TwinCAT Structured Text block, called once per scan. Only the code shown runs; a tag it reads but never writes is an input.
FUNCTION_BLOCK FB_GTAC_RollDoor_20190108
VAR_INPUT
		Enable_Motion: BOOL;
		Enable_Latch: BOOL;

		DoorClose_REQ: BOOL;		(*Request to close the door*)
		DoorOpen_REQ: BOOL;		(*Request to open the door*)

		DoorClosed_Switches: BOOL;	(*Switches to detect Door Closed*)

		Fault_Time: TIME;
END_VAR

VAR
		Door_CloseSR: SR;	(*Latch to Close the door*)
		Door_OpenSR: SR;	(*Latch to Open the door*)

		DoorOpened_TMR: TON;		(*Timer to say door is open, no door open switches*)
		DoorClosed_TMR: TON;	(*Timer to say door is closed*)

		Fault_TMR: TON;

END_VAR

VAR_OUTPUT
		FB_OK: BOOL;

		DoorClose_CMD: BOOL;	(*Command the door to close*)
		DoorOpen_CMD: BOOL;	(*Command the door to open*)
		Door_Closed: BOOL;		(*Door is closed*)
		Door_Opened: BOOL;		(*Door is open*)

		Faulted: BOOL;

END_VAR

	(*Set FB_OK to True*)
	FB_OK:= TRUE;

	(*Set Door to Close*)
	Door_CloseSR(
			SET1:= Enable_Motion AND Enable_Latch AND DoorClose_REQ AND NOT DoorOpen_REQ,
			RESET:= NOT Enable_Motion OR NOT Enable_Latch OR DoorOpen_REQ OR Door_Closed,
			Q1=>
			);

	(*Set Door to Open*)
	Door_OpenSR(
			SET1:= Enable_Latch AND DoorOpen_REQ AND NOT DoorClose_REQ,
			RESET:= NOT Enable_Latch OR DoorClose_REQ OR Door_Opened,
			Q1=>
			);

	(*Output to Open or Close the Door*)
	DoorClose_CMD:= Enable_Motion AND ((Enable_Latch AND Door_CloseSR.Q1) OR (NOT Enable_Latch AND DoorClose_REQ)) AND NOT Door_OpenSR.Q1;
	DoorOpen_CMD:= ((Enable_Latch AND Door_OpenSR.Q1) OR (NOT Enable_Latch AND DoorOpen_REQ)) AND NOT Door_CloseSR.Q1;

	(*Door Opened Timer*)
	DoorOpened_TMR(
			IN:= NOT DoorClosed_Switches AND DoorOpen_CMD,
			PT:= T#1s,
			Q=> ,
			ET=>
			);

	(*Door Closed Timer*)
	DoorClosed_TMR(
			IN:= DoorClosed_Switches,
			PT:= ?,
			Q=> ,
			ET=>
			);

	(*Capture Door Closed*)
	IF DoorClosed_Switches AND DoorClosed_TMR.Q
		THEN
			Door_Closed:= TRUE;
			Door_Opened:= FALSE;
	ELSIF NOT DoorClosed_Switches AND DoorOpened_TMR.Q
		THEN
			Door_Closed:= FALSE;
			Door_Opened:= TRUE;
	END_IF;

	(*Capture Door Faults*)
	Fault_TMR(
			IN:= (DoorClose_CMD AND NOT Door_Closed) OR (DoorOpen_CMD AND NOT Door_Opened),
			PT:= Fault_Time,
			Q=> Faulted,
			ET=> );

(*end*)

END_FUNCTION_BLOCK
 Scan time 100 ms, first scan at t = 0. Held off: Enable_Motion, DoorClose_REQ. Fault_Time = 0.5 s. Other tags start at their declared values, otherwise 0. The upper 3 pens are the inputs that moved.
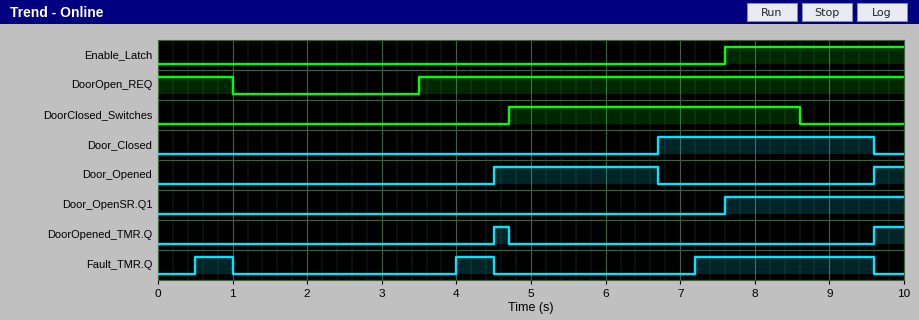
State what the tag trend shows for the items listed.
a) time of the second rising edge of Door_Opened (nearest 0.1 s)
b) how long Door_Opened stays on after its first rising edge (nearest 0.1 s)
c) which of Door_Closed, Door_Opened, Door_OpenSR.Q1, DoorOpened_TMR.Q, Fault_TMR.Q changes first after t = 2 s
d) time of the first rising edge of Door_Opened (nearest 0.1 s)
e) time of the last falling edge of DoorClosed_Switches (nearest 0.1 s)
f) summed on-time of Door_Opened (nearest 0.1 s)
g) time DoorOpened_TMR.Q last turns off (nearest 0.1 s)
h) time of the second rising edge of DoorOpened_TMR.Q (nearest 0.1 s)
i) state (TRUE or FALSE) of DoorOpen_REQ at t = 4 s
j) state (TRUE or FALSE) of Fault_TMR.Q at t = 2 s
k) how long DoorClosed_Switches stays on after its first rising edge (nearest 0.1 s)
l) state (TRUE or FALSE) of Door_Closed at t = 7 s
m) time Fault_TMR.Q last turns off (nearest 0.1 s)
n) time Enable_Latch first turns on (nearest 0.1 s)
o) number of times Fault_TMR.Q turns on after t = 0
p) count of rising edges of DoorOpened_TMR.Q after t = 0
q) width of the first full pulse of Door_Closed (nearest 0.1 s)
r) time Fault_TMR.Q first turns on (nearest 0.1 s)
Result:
9.6 s
2.2 s
Fault_TMR.Q
4.5 s
8.6 s
2.6 s
4.7 s
9.6 s
TRUE
FALSE
3.9 s
TRUE
9.6 s
7.6 s
3
2
2.9 s
0.5 s
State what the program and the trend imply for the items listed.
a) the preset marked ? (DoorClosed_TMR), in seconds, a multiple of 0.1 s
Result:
2.0 s
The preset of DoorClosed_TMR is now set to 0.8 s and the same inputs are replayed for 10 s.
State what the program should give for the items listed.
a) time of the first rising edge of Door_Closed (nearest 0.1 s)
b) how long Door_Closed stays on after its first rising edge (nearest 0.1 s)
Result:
5.5 s
4.1 s
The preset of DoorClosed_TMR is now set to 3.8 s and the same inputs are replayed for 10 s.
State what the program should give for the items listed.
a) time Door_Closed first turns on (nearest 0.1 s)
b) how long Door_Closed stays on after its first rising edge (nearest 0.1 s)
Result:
8.5 s
1.1 s
